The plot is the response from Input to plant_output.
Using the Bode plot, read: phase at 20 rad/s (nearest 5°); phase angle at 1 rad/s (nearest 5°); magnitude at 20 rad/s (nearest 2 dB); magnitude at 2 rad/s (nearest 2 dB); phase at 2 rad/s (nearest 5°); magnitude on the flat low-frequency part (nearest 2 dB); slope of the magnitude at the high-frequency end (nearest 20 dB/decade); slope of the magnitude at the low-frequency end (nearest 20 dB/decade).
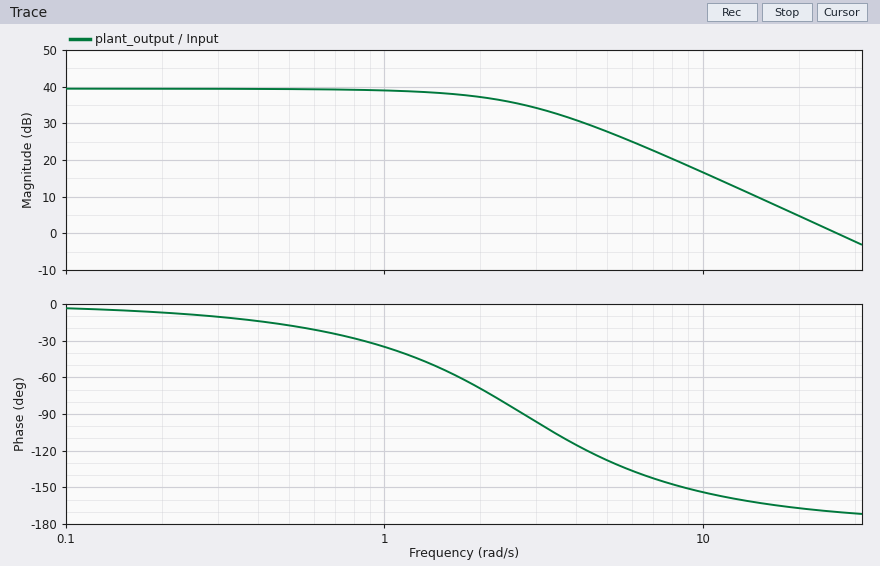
-165°
-35°
4 dB
38 dB
-70°
40 dB
-40 dB/decade
0 dB/decade
